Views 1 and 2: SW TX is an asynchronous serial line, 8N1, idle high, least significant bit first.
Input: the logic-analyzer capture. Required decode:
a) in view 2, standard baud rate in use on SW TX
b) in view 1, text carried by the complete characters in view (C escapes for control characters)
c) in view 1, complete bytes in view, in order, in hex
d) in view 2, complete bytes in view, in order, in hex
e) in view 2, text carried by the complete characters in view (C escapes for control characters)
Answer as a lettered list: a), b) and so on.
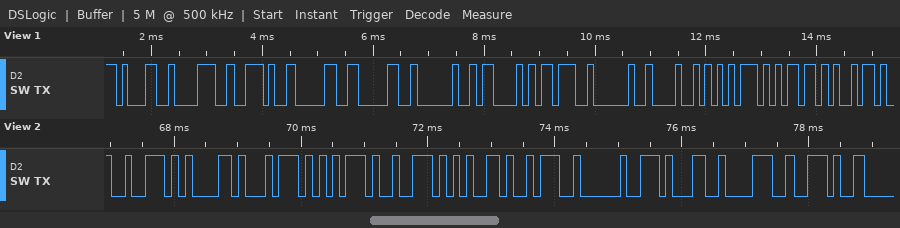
a) 9600 baud
b) "18.00 C; Humi"
c) 31 38 2E 30 30 20 43 3B 20 48 75 6D 69
d) 72 61 74 75 72 65 3A 20 31 38 2E
e) "rature: 18."
